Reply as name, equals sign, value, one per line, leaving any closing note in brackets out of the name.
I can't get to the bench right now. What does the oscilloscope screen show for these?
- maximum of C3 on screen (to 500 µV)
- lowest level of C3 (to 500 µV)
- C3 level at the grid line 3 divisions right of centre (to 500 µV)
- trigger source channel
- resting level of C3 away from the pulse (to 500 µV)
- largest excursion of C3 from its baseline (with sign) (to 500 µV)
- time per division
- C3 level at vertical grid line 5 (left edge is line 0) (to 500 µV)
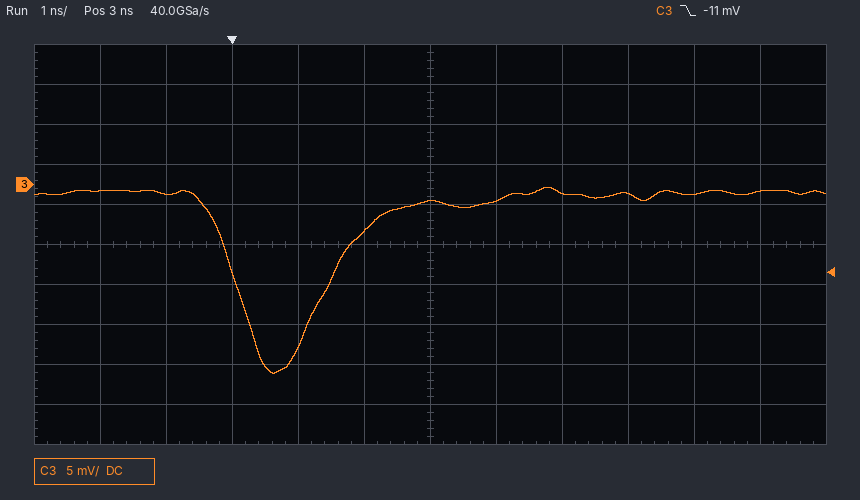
maximum of C3 on screen = -500 µV
lowest level of C3 = -23.5 mV
C3 level at the grid line 3 divisions right of centre = -1.0 mV
trigger source channel = C3
resting level of C3 away from the pulse = -1.0 mV
largest excursion of C3 from its baseline (with sign) = -22.5 mV
time per division = 1 ns
C3 level at vertical grid line 5 (left edge is line 0) = -6.0 mV
